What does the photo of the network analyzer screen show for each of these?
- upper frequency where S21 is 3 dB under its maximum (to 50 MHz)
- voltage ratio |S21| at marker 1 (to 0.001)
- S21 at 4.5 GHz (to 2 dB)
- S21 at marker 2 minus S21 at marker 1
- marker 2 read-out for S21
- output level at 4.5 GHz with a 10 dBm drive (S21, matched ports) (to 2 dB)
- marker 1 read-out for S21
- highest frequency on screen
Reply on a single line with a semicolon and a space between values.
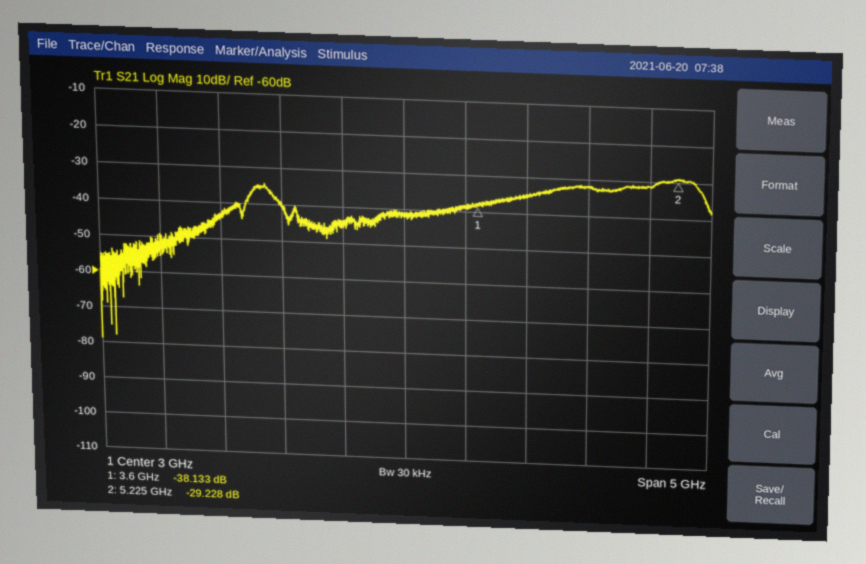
5.40 GHz; 0.012; -32 dB; 8.905 dB; -29.228 dB; -22 dBm; -38.133 dB; 5.5 GHz
